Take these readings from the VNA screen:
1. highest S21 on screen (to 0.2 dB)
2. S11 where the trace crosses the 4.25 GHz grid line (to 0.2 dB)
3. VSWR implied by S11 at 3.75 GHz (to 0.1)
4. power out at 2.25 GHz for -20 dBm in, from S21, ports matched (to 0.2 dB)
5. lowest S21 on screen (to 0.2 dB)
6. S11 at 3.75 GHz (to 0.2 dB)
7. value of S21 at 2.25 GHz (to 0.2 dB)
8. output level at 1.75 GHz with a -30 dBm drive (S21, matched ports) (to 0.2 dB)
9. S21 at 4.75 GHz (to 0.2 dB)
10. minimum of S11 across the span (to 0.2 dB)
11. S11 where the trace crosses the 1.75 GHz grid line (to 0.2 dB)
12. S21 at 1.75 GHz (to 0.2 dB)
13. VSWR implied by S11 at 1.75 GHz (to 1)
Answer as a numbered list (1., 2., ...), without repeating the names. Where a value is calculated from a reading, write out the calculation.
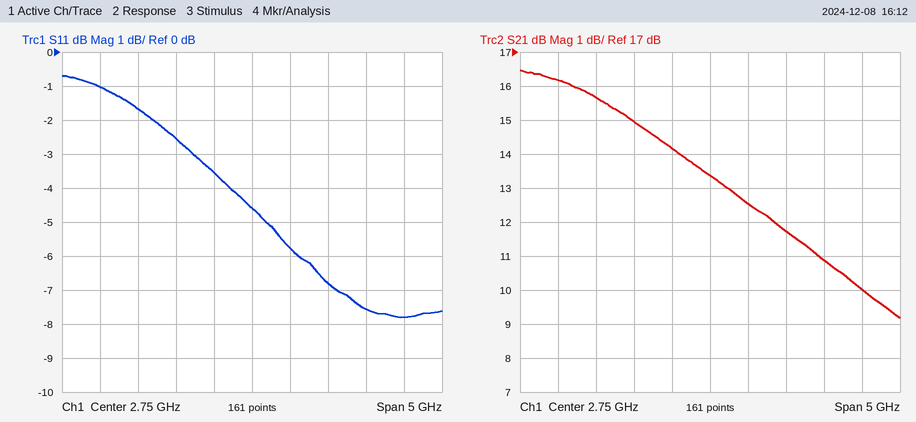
1. 16.4 dB
2. -7.6 dB
3. |Γ| = 10^(-6.8/20) = 0.4571; VSWR = (1 + 0.4571)/(1 − 0.4571) ≈ 2.7
4. -20 dBm + (14.2 dB) = -5.8 dBm
5. 9.2 dB
6. -6.8 dB
7. 14.2 dB
8. -30 dBm + (15.0 dB) = -15.0 dBm
9. 10.0 dB
10. -7.8 dB
11. -2.6 dB
12. 15.0 dB
13. |Γ| = 10^(-2.6/20) = 0.7413; VSWR = (1 + 0.7413)/(1 − 0.7413) ≈ 7
